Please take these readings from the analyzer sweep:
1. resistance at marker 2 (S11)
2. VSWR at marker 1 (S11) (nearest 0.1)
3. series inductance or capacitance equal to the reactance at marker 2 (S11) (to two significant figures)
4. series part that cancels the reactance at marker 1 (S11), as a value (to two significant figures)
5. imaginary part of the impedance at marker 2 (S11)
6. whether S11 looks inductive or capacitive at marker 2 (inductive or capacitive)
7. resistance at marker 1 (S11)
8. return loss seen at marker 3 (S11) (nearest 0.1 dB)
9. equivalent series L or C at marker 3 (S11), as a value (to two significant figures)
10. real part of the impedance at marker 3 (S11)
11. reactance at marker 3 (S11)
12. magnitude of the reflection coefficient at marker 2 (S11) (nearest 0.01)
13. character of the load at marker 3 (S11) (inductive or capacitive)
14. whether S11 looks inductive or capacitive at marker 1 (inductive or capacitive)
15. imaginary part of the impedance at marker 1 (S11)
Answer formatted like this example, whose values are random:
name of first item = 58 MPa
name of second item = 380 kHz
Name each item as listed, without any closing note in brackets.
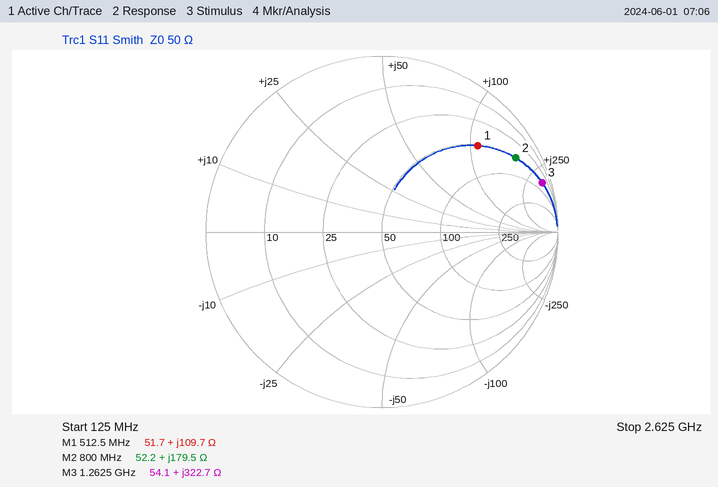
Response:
resistance at marker 2 = 52.2 Ω
VSWR at marker 1 (S11) = 6.5
series inductance or capacitance equal to the reactance at marker 2 (S11) = 36 nH
series part that cancels the reactance at marker 1 (S11), as a value = 2.8 pF
imaginary part of the impedance at marker 2 = +179.5 Ω
whether S11 looks inductive or capacitive at marker 2 = inductive
resistance at marker 1 = 51.7 Ω
return loss seen at marker 3 (S11) = 0.4 dB
equivalent series L or C at marker 3 (S11), as a value = 41 nH
real part of the impedance at marker 3 = 54.1 Ω
reactance at marker 3 = +322.7 Ω
magnitude of the reflection coefficient at marker 2 (S11) = 0.87
character of the load at marker 3 (S11) = inductive
whether S11 looks inductive or capacitive at marker 1 = inductive
imaginary part of the impedance at marker 1 = +109.7 Ω
